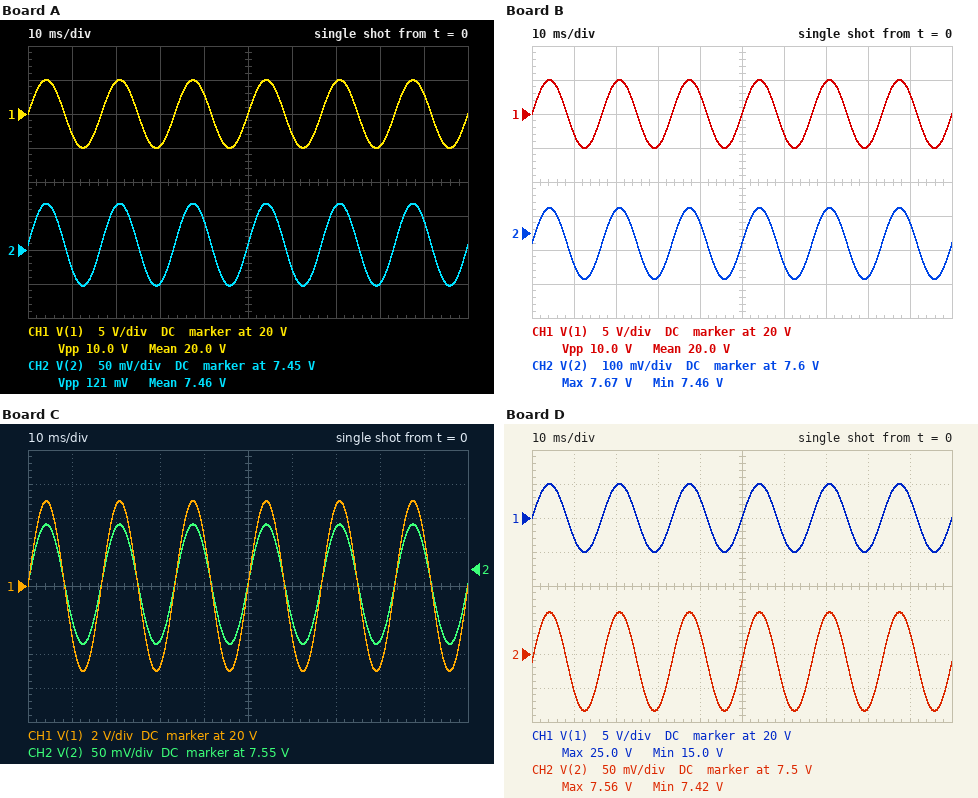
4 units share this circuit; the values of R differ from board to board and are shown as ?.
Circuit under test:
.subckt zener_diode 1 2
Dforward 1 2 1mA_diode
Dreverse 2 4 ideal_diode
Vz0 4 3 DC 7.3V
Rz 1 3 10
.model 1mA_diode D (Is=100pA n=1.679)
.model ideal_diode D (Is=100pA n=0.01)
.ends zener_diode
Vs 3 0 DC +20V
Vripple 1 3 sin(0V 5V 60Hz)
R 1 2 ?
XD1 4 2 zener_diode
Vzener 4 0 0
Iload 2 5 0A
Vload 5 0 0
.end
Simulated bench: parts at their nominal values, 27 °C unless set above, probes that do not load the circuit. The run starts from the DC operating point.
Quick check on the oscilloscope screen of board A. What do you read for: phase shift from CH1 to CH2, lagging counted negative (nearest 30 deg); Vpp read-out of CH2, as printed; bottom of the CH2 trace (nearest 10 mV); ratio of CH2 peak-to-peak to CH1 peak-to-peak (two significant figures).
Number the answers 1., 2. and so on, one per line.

1. 0 deg
2. 121 mV
3. 7.40 V
4. 0.012
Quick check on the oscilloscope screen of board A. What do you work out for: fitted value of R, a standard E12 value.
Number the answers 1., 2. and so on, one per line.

1. 820 Ω
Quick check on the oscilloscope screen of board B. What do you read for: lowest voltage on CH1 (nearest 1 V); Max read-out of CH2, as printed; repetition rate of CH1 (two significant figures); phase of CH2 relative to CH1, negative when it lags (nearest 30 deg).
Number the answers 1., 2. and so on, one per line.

1. 15 V
2. 7.67 V
3. 60 Hz
4. 0 deg
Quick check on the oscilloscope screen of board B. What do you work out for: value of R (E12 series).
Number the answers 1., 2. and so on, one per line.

1. 470 Ω
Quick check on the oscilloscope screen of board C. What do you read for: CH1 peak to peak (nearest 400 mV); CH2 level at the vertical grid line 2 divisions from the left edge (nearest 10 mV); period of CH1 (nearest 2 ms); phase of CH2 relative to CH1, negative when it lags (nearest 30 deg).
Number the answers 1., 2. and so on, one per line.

1. 10.0 V
2. 7.61 V
3. 16 ms
4. 0 deg
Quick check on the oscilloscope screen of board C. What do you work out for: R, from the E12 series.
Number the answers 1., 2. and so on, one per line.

1. 560 Ω
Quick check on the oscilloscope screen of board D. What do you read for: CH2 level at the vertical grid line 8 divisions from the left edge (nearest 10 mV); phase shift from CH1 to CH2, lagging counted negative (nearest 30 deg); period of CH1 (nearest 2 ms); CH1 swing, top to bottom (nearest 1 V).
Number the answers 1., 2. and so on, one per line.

1. 7.42 V
2. 0 deg
3. 16 ms
4. 10 V
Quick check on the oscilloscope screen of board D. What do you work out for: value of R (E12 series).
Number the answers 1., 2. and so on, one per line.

1. 680 Ω
